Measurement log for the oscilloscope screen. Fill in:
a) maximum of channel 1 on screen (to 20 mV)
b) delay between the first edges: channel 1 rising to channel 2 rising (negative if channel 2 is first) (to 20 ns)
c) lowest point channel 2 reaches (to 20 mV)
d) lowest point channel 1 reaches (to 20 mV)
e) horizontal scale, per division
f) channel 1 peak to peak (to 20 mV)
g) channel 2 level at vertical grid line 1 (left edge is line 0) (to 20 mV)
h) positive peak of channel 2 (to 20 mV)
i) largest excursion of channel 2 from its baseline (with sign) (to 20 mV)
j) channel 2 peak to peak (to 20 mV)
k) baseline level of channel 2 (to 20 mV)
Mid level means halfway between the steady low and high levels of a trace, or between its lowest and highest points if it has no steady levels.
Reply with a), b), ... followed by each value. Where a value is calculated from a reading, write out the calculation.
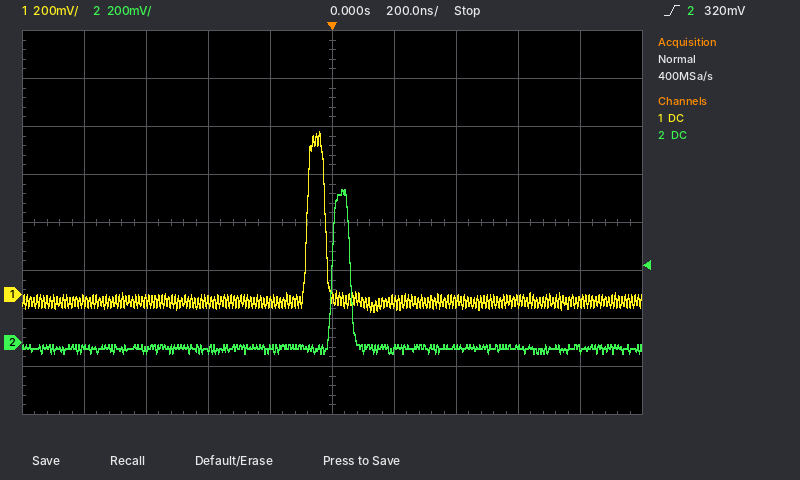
a) 680 mV
b) +80 ns
c) -40 mV
d) -80 mV
e) 200 ns
f) 680 mV − (-80 mV) = 760 mV
g) -20 mV
h) 640 mV
i) 640 mV − (-20 mV) = +660 mV
j) 640 mV − (-40 mV) = 680 mV
k) -20 mV
